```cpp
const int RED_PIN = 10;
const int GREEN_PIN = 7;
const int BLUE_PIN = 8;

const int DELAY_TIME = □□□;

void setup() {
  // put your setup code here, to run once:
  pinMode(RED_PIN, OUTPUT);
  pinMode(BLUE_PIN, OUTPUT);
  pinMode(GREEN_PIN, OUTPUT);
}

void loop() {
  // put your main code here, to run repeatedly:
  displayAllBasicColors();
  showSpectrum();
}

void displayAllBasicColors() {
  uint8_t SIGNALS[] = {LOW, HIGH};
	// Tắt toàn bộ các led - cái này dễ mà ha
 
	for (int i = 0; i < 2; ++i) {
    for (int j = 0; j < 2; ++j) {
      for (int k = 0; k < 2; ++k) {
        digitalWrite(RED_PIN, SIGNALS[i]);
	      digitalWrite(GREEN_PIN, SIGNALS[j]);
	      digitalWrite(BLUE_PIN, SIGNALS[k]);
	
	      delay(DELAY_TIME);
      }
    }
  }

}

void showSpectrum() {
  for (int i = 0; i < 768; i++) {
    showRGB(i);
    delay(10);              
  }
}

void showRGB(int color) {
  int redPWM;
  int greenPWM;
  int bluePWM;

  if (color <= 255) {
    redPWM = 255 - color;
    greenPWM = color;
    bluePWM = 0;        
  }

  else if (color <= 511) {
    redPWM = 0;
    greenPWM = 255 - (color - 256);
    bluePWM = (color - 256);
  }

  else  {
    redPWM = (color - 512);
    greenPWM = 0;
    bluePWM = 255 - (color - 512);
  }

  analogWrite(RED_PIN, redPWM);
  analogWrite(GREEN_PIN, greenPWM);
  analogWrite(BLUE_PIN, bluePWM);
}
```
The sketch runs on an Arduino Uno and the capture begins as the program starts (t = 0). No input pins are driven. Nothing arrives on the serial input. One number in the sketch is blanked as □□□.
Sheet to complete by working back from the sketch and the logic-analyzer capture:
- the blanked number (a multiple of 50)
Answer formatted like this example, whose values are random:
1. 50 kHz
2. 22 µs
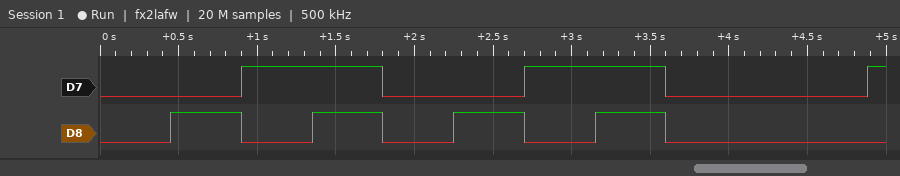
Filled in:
1. 450
